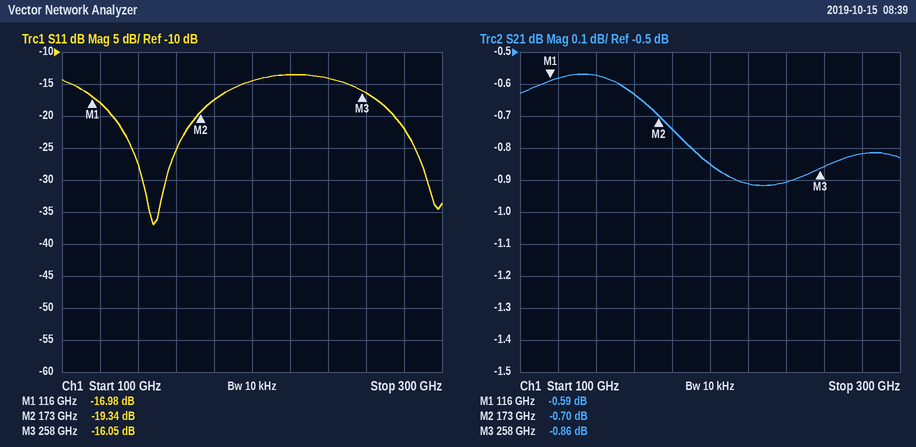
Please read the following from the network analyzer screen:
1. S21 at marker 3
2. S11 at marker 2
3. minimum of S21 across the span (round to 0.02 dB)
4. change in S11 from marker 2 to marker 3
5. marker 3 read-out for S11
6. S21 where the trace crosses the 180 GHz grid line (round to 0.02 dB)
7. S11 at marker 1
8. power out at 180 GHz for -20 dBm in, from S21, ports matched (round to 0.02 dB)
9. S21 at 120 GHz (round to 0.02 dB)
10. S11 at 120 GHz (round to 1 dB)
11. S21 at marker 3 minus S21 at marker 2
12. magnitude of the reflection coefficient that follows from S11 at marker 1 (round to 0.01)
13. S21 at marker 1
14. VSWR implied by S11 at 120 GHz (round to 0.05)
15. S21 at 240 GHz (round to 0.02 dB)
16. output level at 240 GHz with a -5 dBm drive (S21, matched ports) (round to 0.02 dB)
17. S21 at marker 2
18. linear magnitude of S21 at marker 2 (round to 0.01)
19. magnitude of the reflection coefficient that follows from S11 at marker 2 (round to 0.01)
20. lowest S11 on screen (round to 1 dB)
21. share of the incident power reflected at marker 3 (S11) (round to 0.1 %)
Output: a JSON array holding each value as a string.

["-0.86 dB", "-19.34 dB", "-0.92 dB", "3.29 dB", "-16.05 dB", "-0.74 dB", "-16.98 dB", "-20.74 dBm", "-0.58 dB", "-18 dB", "-0.16 dB", "0.14", "-0.59 dB", "1.30", "-0.90 dB", "-5.90 dBm", "-0.70 dB", "0.92", "0.11", "-37 dB", "2.5 %"]
